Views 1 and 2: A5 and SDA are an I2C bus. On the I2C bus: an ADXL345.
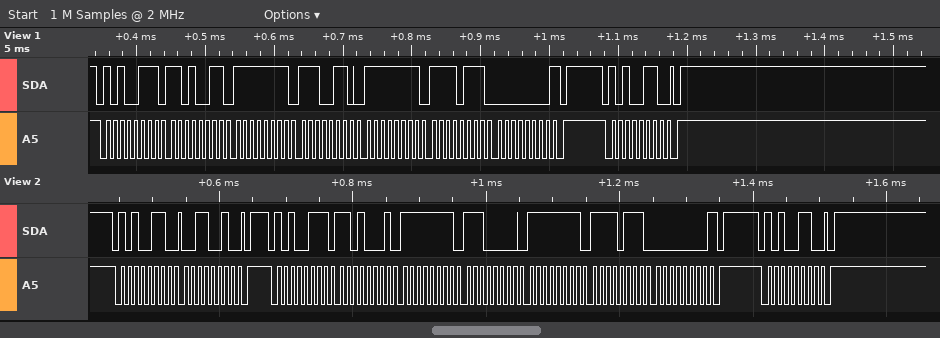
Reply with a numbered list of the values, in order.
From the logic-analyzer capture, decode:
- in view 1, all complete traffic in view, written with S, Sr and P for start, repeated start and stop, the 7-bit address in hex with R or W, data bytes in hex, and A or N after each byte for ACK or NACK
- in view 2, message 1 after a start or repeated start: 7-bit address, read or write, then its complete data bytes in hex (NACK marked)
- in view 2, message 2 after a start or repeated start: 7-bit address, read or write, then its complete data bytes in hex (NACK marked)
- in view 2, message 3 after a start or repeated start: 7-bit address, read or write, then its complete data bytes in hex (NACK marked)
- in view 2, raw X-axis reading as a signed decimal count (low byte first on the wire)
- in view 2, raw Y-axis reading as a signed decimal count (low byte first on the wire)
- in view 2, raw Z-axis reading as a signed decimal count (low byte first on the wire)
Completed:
1. S 53R A D3 A FF A E6 A FF A F7 A 00 N P S 53W A P
2. 0x53 write: 32
3. 0x53 read: D1 FF E0 FF F7 00 NACK
4. 0x53 write
5. -47
6. -32
7. 247
